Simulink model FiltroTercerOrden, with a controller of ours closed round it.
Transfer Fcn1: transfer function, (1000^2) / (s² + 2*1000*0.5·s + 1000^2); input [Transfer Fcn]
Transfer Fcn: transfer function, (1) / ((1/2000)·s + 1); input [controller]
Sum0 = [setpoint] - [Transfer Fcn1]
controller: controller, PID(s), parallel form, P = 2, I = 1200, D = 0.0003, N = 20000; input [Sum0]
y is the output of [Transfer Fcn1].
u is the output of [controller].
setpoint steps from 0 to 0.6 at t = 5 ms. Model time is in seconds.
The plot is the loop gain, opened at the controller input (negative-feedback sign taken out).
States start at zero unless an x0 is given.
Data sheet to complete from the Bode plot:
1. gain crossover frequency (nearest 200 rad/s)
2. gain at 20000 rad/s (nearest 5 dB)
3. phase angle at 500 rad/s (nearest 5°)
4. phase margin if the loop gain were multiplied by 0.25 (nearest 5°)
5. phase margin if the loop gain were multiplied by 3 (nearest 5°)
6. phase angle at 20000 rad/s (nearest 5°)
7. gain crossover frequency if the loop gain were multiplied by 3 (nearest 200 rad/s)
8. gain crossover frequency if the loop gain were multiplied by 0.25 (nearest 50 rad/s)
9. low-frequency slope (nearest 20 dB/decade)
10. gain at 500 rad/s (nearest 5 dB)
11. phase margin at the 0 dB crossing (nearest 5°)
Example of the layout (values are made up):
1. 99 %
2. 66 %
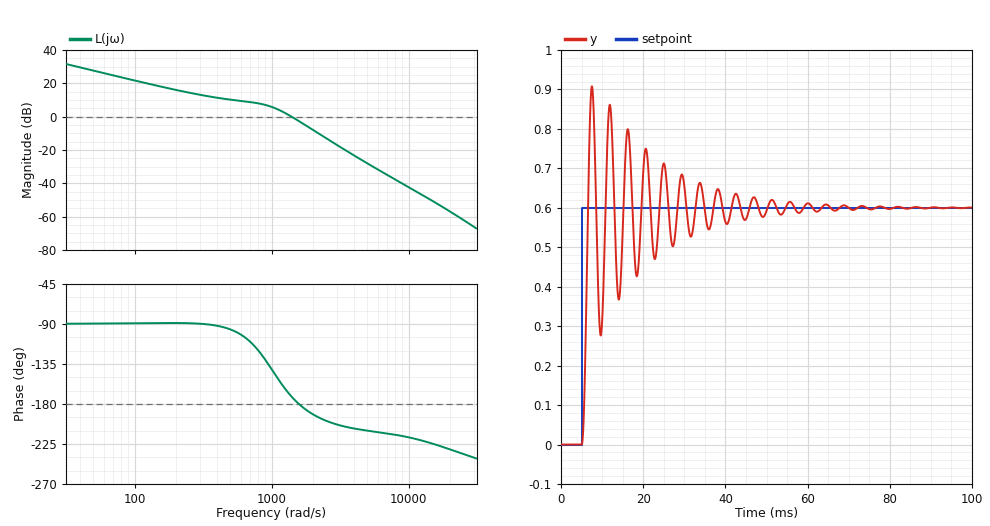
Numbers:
1. 1400 rad/s
2. -55 dB
3. -95°
4. 90°
5. -15°
6. -230°
7. 2200 rad/s
8. 350 rad/s
9. -20 dB/decade
10. 10 dB
11. 10°
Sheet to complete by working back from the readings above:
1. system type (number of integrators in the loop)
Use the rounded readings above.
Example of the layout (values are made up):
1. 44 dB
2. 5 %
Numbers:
1. 1
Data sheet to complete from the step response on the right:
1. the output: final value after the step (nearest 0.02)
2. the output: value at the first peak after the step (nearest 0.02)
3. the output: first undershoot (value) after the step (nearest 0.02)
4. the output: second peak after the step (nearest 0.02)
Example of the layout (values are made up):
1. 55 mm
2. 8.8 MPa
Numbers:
1. 0.60
2. 0.90
3. 0.28
4. 0.86
